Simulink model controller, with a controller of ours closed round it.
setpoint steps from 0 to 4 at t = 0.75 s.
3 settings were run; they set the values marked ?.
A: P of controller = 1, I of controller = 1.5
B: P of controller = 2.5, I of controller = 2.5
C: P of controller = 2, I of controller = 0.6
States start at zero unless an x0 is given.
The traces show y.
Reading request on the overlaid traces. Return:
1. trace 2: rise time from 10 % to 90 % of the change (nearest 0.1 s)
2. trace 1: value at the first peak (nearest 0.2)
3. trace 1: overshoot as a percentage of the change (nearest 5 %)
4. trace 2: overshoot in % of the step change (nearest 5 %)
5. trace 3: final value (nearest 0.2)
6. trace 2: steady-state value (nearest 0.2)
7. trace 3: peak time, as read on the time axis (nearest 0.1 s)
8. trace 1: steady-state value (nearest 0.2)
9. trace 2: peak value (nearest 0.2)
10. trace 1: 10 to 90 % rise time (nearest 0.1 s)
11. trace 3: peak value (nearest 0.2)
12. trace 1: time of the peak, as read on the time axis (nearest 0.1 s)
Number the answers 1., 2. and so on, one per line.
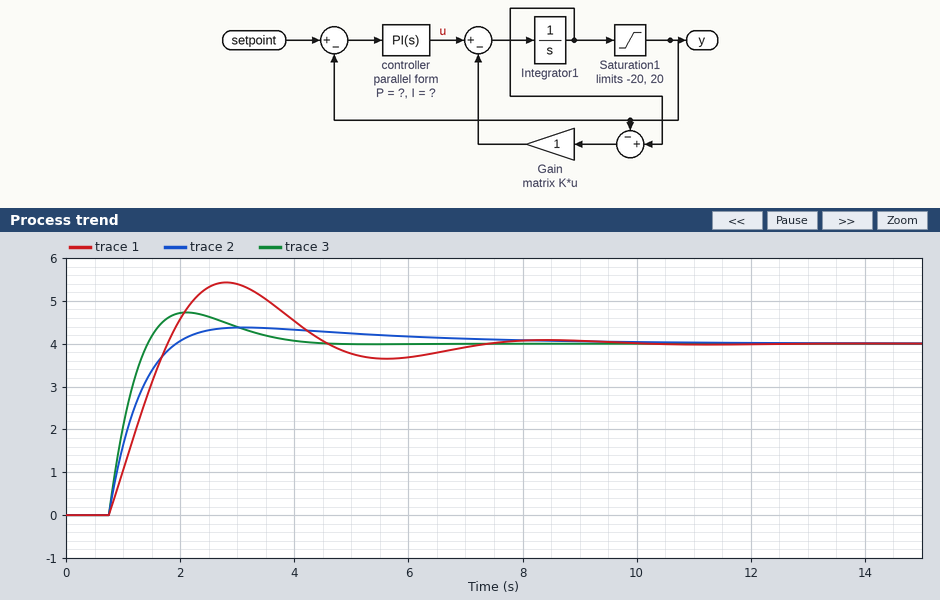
1. 0.8 s
2. 5.4
3. 35 %
4. 10 %
5. 4.0
6. 4.0
7. 2.1 s
8. 4.0
9. 4.4
10. 0.8 s
11. 4.8
12. 2.8 s
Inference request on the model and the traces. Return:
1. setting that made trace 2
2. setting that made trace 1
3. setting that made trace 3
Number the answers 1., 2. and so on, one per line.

1. C
2. A
3. B
